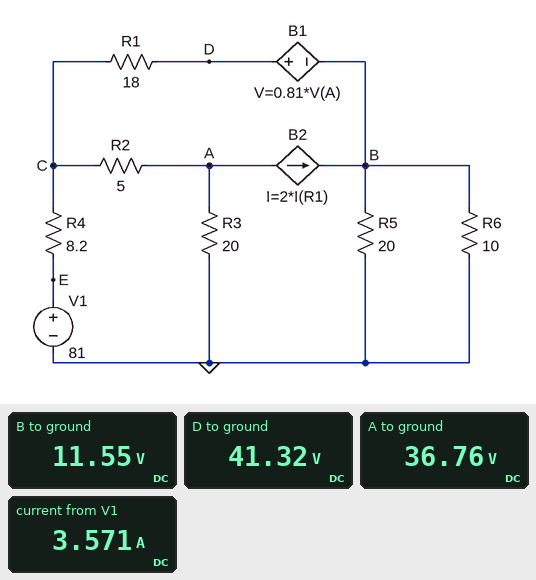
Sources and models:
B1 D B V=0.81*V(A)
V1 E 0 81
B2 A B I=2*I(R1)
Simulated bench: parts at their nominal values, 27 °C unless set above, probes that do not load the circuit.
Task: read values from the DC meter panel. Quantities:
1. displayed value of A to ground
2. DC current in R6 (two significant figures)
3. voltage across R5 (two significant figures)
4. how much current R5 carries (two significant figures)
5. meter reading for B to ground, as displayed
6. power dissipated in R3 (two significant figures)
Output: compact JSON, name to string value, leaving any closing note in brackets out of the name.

{"displayed value of A to ground": "36.76 V", "DC current in R6": "1.2 A", "voltage across R5": "12 V", "how much current R5 carries": "580 mA", "meter reading for B to ground, as displayed": "11.55 V", "power dissipated in R3": "68 W"}
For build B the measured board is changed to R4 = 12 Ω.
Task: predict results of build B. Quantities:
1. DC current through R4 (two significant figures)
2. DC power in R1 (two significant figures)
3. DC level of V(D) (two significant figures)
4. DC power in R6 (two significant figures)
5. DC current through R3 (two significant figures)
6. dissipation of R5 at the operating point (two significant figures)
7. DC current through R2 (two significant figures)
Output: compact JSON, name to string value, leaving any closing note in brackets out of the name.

{"DC current through R4": "3.1 A", "DC power in R1": "4.4 W", "DC level of V(D)": "35 V", "DC power in R6": "9.8 W", "DC current through R3": "1.6 A", "dissipation of R5 at the operating point": "4.9 W", "DC current through R2": "2.6 A"}
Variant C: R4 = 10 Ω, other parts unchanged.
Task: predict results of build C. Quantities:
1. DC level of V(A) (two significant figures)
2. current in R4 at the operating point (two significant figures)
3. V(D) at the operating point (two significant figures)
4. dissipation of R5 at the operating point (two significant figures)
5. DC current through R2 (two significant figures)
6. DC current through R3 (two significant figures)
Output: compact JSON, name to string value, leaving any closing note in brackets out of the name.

{"DC level of V(A)": "34 V", "current in R4 at the operating point": "3.3 A", "V(D) at the operating point": "38 V", "dissipation of R5 at the operating point": "5.7 W", "DC current through R2": "2.8 A", "DC current through R3": "1.7 A"}
